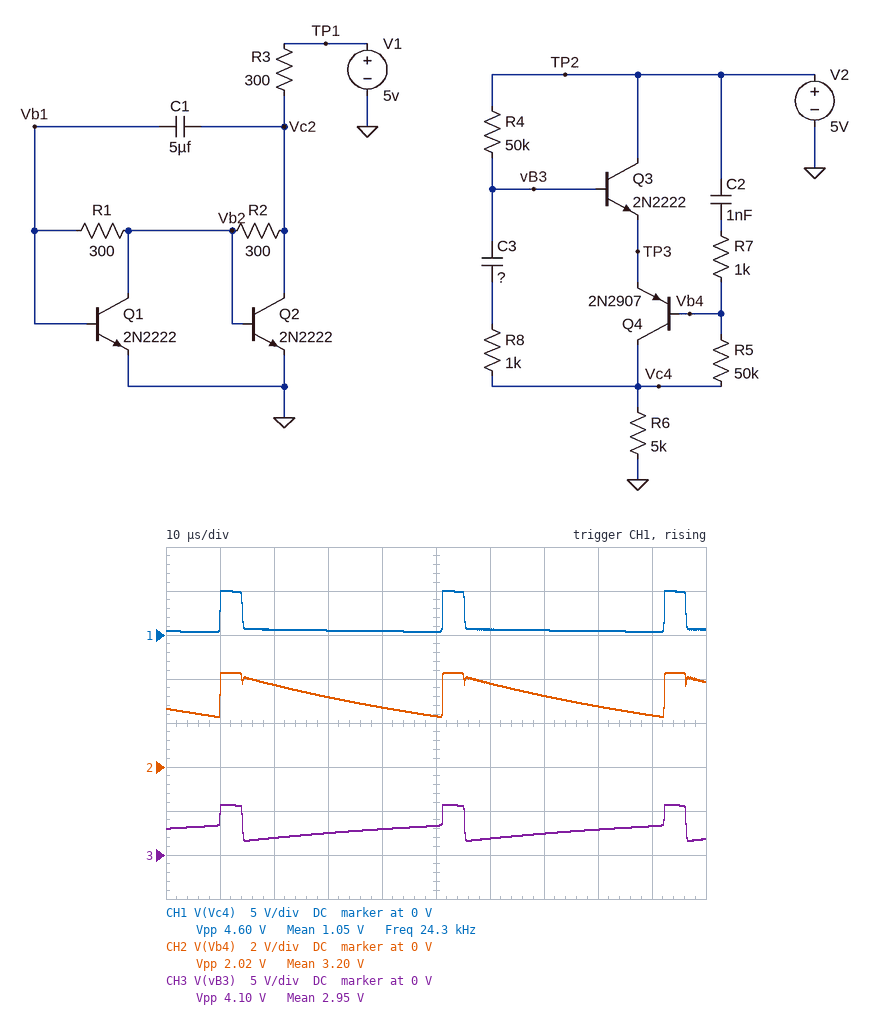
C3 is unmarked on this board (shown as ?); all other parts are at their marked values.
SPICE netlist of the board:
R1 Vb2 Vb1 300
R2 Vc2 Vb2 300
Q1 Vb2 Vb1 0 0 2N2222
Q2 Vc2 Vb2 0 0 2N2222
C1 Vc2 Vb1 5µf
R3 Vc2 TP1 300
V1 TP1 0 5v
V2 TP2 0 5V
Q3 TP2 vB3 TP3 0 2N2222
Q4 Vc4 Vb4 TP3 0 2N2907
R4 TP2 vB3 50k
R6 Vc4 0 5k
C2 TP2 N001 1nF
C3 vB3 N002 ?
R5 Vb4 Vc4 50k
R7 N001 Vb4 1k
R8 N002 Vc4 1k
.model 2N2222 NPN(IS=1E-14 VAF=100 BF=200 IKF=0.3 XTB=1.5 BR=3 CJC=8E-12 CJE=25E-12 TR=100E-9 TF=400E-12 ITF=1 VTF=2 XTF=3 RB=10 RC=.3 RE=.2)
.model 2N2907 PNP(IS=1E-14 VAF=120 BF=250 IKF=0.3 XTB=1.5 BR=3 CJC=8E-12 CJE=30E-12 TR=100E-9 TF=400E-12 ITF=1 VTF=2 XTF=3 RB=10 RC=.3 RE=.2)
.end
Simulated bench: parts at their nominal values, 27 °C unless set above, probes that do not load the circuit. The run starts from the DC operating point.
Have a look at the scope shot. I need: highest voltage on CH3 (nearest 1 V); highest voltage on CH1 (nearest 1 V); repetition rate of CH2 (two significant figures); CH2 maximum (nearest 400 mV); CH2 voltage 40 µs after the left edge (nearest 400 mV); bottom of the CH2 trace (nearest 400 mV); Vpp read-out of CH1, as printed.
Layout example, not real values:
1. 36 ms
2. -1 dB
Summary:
1. 6 V
2. 5 V
3. 24 kHz
4. 4.4 V
5. 2.8 V
6. 2.4 V
7. 4.60 V
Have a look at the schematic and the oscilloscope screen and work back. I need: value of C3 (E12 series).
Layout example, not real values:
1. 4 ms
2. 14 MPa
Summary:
1. 820 pF
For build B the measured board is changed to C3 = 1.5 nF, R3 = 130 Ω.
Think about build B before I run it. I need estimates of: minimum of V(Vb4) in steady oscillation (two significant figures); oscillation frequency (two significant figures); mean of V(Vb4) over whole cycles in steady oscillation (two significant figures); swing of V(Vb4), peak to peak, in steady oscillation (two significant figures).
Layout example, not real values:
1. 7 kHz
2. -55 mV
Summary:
1. 1.9 V
2. 18 kHz
3. 3.0 V
4. 2.4 V
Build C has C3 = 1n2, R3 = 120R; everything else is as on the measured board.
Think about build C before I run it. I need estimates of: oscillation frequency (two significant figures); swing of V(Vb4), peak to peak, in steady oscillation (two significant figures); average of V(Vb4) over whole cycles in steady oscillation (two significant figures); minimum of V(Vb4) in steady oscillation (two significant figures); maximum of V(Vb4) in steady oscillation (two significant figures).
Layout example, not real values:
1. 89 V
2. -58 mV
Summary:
1. 20 kHz
2. 2.3 V
3. 3.1 V
4. 2.0 V
5. 4.3 V
